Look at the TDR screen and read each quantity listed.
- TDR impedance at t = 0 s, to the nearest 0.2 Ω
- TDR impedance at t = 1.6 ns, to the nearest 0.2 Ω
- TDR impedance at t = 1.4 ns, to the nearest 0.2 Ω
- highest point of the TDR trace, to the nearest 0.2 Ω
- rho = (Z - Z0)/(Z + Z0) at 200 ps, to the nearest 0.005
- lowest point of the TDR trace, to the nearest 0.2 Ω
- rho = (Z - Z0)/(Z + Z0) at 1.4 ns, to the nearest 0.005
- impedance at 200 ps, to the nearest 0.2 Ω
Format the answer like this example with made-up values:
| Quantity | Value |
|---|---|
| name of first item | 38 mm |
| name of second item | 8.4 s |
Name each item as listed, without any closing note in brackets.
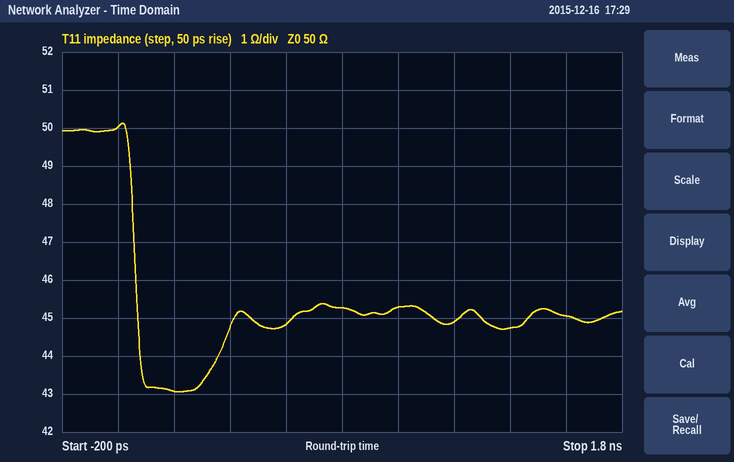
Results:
| Quantity | Value |
|---|---|
| TDR impedance at t = 0 s, to the nearest 0.2 Ω | 50.0 Ω |
| TDR impedance at t = 1.6 ns, to the nearest 0.2 Ω | 45.0 Ω |
| TDR impedance at t = 1.4 ns, to the nearest 0.2 Ω | 44.8 Ω |
| highest point of the TDR trace, to the nearest 0.2 Ω | 50.2 Ω |
| rho = (Z - Z0)/(Z + Z0) at 200 ps, to the nearest 0.005 | -0.075 |
| lowest point of the TDR trace, to the nearest 0.2 Ω | 43.0 Ω |
| rho = (Z - Z0)/(Z + Z0) at 1.4 ns, to the nearest 0.005 | -0.055 |
| impedance at 200 ps, to the nearest 0.2 Ω | 43.0 Ω |
